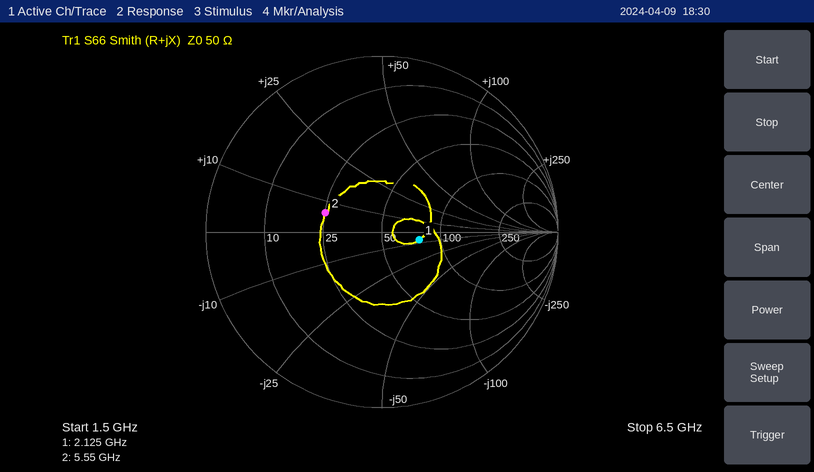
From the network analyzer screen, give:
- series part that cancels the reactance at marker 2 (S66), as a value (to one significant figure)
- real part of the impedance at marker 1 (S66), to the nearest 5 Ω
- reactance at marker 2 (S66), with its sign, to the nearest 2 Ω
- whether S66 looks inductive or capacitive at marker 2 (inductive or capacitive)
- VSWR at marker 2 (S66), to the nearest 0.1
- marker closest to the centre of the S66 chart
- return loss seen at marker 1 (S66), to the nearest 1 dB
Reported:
5 pF
75 Ω
+6 Ω
inductive
2.0
marker 1
13 dB
